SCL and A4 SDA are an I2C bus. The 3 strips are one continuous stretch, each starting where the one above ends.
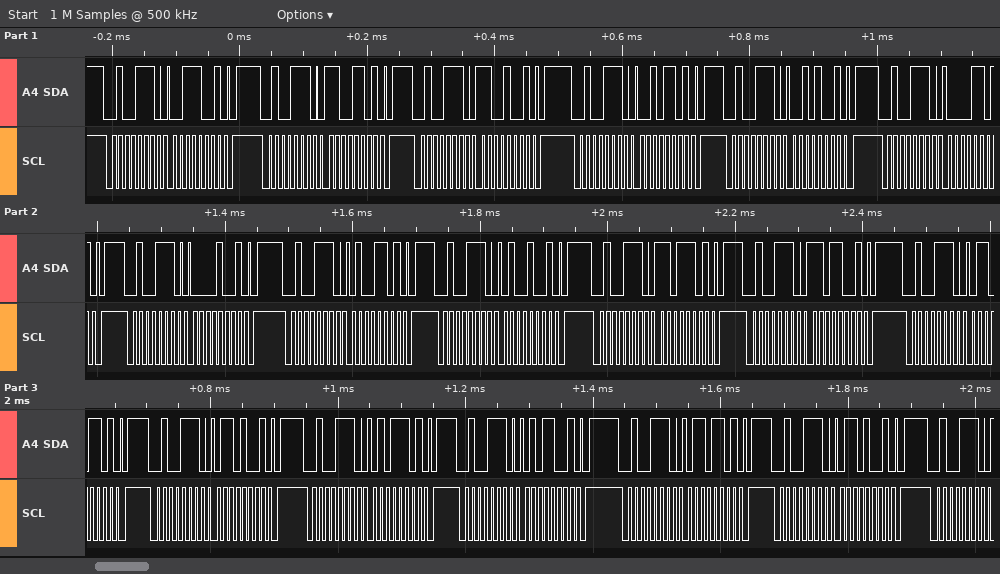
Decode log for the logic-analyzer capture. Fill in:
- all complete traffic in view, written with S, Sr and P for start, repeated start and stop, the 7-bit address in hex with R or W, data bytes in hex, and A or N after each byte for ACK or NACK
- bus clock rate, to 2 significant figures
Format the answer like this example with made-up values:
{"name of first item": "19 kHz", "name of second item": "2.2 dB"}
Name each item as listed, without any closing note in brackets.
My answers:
{"all complete traffic in view, written with S, Sr and P for start, repeated start and stop, the 7-bit address in hex with R or W, data bytes in hex, and A or N after each byte for ACK or NACK": "S 27W A 39 A P S 27W A CD A P S 27W A C9 A P S 27W A 2D A P S 27W A 29 A P S 27W A 0D A P S 27W A 09 A P S 27W A 4D A P S 27W A 49 A P S 27W A DD A P S 27W A D9 A P S 27W A 6D A P S 27W A 69 A P S 27W A 5D A P S 27W A 59 A P S 27W A 6D A P S 27W A 69 A P S 27W A", "bus clock rate, to 2 significant figures": "100 kHz"}
